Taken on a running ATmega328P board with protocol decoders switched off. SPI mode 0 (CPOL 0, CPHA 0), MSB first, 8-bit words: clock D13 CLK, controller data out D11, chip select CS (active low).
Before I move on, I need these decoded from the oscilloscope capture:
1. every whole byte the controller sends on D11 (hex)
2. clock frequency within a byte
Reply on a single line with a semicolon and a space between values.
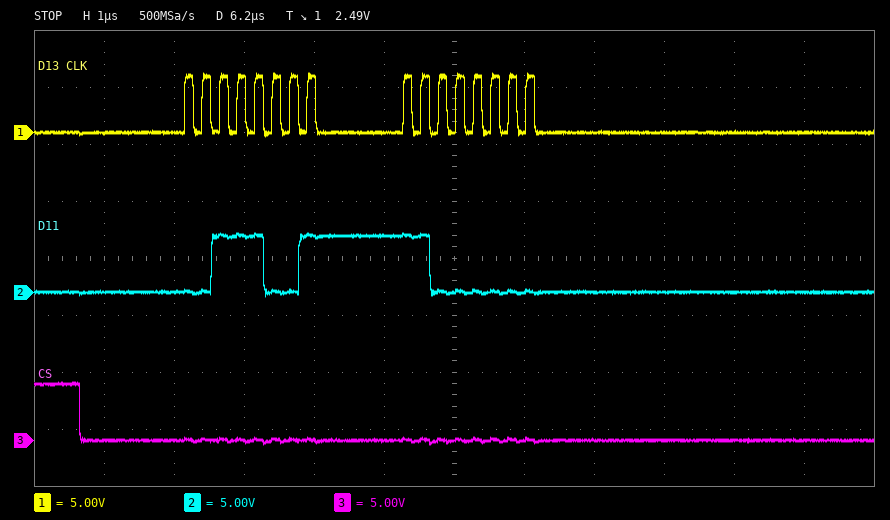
39 C0; 4 MHz
